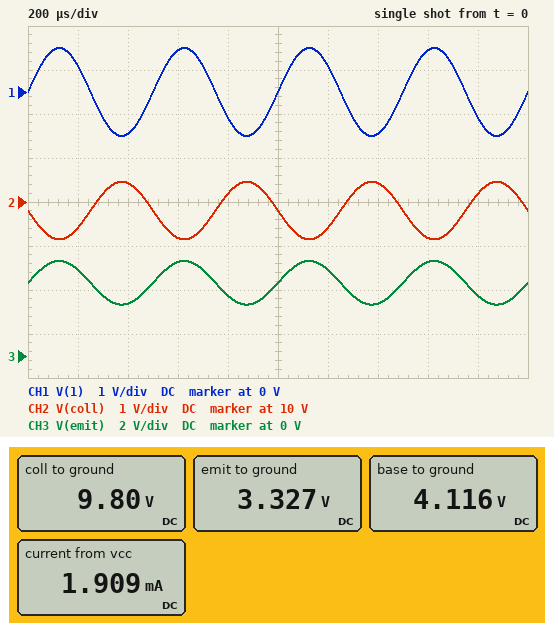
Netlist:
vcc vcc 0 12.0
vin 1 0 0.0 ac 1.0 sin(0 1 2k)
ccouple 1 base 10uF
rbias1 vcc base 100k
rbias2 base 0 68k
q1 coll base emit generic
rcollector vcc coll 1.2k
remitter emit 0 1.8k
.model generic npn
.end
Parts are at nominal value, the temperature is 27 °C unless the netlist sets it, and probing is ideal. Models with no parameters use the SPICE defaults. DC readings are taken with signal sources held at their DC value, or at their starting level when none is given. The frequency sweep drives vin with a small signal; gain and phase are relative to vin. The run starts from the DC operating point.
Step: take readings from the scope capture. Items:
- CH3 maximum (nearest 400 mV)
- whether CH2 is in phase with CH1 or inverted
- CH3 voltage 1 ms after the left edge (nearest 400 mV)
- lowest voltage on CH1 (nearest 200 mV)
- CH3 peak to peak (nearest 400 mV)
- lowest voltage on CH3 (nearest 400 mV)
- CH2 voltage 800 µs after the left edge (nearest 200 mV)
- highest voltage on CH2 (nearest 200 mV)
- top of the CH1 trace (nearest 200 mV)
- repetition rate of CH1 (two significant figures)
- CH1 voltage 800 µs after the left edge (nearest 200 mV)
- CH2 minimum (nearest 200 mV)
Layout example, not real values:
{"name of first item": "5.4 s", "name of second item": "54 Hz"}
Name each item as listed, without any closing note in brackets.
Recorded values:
{"CH3 maximum": "4.4 V", "whether CH2 is in phase with CH1 or inverted": "inverted", "CH3 voltage 1 ms after the left edge": "3.2 V", "lowest voltage on CH1": "-1.0 V", "CH3 peak to peak": "2.0 V", "lowest voltage on CH3": "2.4 V", "CH2 voltage 800 µs after the left edge": "10.2 V", "highest voltage on CH2": "10.4 V", "top of the CH1 trace": "1.0 V", "repetition rate of CH1": "2.0 kHz", "CH1 voltage 800 µs after the left edge": "-600 mV", "CH2 minimum": "9.2 V"}
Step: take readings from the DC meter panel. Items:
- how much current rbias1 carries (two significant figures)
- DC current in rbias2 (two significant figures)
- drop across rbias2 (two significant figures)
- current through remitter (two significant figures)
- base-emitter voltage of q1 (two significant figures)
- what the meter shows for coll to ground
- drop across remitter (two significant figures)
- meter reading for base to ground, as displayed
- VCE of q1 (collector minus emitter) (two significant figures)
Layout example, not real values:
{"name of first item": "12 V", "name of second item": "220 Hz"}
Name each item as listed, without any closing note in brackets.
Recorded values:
{"how much current rbias1 carries": "79 µA", "DC current in rbias2": "61 µA", "drop across rbias2": "4.1 V", "current through remitter": "1.8 mA", "base-emitter voltage of q1": "790 mV", "what the meter shows for coll to ground": "9.80 V", "drop across remitter": "3.3 V", "meter reading for base to ground, as displayed": "4.116 V", "VCE of q1 (collector minus emitter)": "6.5 V"}
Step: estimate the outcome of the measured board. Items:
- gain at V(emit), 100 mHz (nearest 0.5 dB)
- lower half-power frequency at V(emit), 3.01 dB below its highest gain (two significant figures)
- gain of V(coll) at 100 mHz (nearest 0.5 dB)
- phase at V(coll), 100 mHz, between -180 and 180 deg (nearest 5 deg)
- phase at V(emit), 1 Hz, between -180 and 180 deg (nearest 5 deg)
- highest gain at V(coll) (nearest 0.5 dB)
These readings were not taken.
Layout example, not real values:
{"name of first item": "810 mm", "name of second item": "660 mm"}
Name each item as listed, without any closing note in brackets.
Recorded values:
{"gain at V(emit), 100 mHz": "-14.0 dB", "lower half-power frequency at V(emit), 3.01 dB below its highest gain": "480 mHz", "gain of V(coll) at 100 mHz": "-17.5 dB", "phase at V(coll), 100 mHz, between -180 and 180 deg": "-100 deg", "phase at V(emit), 1 Hz, between -180 and 180 deg": "25 deg", "highest gain at V(coll)": "-3.5 dB"}
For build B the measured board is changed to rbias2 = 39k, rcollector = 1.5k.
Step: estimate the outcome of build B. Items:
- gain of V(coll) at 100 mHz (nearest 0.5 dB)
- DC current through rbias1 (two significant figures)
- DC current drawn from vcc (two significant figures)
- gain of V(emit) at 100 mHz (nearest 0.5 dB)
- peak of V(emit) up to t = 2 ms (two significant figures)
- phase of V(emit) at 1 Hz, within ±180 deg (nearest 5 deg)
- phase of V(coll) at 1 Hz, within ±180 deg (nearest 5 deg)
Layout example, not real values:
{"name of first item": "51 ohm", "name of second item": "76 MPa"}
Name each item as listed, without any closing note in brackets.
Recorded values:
{"gain of V(coll) at 100 mHz": "-18.0 dB", "DC current through rbias1": "90 µA", "DC current drawn from vcc": "1.3 mA", "gain of V(emit) at 100 mHz": "-16.5 dB", "peak of V(emit) up to t = 2 ms": "3.2 V", "phase of V(emit) at 1 Hz, within ±180 deg": "35 deg", "phase of V(coll) at 1 Hz, within ±180 deg": "-145 deg"}
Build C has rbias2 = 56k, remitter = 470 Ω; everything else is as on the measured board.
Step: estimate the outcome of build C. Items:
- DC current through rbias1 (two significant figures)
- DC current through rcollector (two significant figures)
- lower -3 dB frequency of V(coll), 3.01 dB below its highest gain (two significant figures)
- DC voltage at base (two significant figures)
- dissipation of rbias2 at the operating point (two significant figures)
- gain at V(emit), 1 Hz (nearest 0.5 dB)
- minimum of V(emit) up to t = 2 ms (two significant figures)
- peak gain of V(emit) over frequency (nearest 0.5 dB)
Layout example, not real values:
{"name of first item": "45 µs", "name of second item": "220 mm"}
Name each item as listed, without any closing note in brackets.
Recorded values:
{"DC current through rbias1": "92 µA", "DC current through rcollector": "4.2 mA", "lower -3 dB frequency of V(coll), 3.01 dB below its highest gain": "770 mHz", "DC voltage at base": "2.8 V", "dissipation of rbias2 at the operating point": "140 µW", "gain at V(emit), 1 Hz": "-2.0 dB", "minimum of V(emit) up to t = 2 ms": "1.0 V", "peak gain of V(emit) over frequency": "0 dB"}
